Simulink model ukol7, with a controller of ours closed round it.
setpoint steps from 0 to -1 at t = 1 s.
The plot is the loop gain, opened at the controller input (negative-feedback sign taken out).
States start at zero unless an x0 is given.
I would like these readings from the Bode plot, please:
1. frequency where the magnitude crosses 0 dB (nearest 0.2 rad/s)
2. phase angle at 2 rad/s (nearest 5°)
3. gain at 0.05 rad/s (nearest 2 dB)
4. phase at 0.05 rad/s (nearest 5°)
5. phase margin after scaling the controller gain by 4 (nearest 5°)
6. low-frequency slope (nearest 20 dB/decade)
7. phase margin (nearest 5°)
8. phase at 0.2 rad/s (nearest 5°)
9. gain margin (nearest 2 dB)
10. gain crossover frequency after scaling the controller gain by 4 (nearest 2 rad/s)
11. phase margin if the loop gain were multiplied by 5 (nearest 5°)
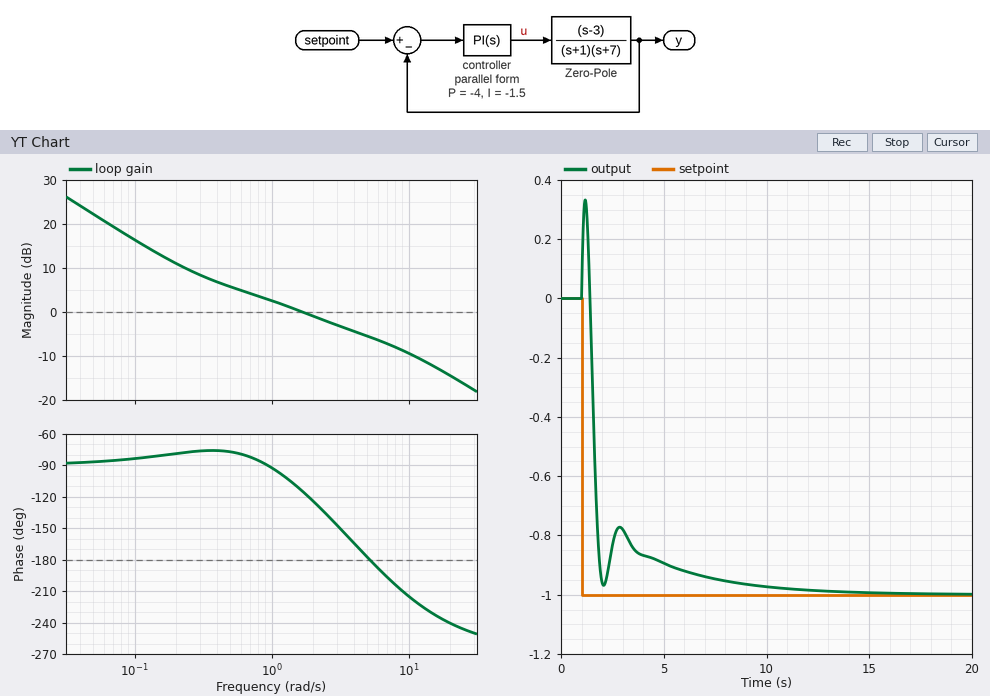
1.6 rad/s
-125°
22 dB
-85°
-50°
-20 dB/decade
65°
-80°
6 dB
14 rad/s
-60°
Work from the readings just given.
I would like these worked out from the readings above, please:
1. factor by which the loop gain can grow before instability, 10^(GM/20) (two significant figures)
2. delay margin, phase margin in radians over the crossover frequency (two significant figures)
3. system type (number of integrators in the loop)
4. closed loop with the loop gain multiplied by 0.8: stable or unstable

2.0
0.71 s
1
stable
